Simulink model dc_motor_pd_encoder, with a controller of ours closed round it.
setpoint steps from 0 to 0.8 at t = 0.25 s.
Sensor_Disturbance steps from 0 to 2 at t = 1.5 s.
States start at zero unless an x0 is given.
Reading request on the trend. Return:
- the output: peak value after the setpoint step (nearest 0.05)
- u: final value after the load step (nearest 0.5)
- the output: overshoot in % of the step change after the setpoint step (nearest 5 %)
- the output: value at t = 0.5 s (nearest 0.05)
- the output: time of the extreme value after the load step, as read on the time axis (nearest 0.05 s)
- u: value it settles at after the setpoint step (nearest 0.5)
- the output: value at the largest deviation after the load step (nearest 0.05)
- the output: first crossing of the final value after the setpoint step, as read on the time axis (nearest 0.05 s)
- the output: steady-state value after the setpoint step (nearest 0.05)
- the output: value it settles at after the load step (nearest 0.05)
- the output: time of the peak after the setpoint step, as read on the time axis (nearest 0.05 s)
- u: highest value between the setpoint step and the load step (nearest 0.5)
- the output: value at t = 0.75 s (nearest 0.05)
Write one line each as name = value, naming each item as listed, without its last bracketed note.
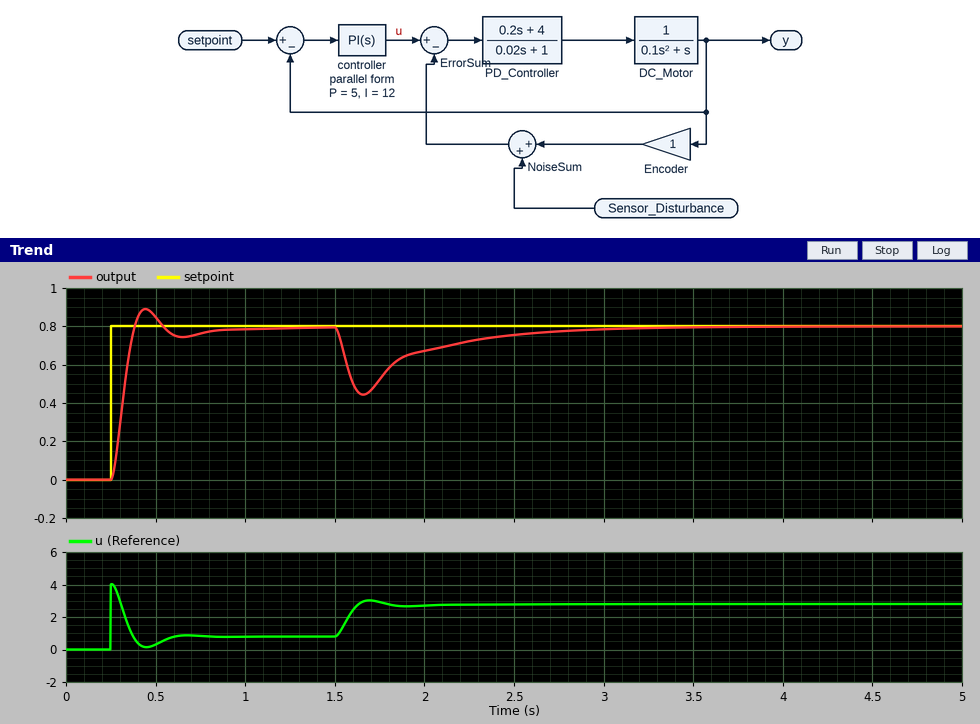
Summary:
the output: peak value after the setpoint step = 0.90
u: final value after the load step = 3.0
the output: overshoot in % of the step change after the setpoint step = 10 %
the output: value at t = 0.5 s = 0.85
the output: time of the extreme value after the load step, as read on the time axis = 1.65 s
u: value it settles at after the setpoint step = 1.0
the output: value at the largest deviation after the load step = 0.45
the output: first crossing of the final value after the setpoint step, as read on the time axis = 0.40 s
the output: steady-state value after the setpoint step = 0.80
the output: value it settles at after the load step = 0.80
the output: time of the peak after the setpoint step, as read on the time axis = 0.45 s
u: highest value between the setpoint step and the load step = 4.0
the output: value at t = 0.75 s = 0.75
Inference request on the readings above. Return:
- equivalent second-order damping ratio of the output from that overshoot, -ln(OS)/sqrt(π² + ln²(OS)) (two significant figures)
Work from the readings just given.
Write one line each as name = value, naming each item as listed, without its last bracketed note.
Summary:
equivalent second-order damping ratio of the output from that overshoot, -ln(OS)/sqrt(π² + ln²(OS)) = 0.59
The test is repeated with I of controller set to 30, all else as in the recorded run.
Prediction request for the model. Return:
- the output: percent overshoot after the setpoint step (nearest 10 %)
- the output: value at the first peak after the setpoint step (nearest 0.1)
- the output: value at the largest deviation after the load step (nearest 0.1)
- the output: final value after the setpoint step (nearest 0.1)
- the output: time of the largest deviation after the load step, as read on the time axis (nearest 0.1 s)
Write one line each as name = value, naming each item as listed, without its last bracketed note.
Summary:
the output: percent overshoot after the setpoint step = 30 %
the output: value at the first peak after the setpoint step = 1.0
the output: value at the largest deviation after the load step = 0.5
the output: final value after the setpoint step = 0.8
the output: time of the largest deviation after the load step, as read on the time axis = 1.6 s
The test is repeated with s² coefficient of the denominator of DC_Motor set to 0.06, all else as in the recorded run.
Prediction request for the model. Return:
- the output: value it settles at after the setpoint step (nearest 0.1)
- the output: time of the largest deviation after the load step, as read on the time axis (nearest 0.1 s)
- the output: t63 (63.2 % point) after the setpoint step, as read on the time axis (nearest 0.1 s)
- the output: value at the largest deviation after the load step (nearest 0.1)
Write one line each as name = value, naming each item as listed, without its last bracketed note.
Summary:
the output: value it settles at after the setpoint step = 0.8
the output: time of the largest deviation after the load step, as read on the time axis = 1.6 s
the output: t63 (63.2 % point) after the setpoint step, as read on the time axis = 0.3 s
the output: value at the largest deviation after the load step = 0.5
